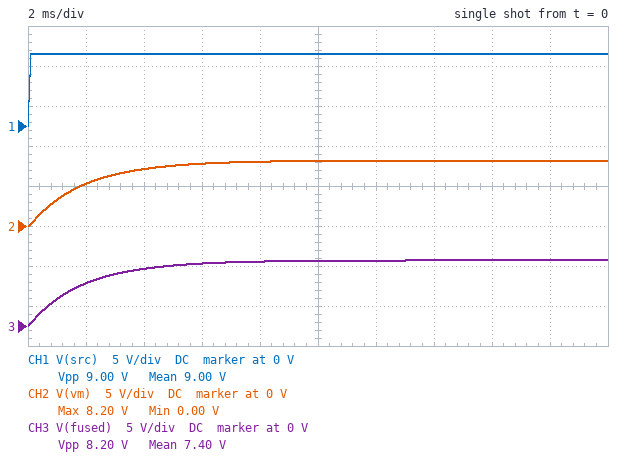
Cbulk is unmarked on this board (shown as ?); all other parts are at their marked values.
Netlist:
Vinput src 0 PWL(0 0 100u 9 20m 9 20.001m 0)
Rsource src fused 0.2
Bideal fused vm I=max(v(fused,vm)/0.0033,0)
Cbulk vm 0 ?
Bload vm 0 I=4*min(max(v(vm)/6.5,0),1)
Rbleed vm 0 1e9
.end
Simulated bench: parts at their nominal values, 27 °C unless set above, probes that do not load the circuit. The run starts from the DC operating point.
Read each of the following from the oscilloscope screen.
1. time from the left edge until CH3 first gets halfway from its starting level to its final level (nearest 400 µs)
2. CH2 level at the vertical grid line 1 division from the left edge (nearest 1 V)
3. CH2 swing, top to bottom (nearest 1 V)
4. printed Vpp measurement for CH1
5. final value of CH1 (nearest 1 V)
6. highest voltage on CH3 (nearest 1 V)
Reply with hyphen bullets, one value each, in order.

- 1.2 ms
- 5 V
- 8 V
- 9.00 V
- 9 V
- 8 V
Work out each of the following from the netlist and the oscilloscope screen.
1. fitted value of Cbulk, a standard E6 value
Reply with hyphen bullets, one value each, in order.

- 10 mF
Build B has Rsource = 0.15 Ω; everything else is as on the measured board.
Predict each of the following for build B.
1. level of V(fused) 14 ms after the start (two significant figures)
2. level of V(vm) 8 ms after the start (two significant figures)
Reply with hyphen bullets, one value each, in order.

- 8.4 V
- 8.3 V
